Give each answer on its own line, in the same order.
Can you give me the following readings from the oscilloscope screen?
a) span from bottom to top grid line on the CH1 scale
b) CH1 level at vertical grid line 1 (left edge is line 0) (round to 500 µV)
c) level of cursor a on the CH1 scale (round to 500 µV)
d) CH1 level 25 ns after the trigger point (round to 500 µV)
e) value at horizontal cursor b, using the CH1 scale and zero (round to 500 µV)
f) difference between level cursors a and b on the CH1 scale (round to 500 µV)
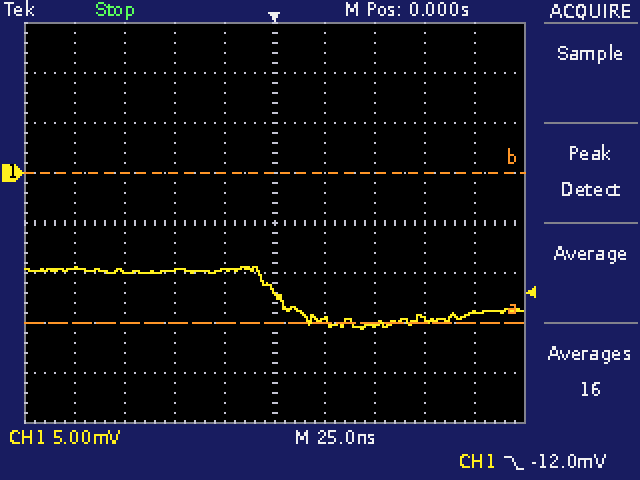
40 mV
-9.5 mV
-15.0 mV
-14.5 mV
0.0 mV
15.0 mV
